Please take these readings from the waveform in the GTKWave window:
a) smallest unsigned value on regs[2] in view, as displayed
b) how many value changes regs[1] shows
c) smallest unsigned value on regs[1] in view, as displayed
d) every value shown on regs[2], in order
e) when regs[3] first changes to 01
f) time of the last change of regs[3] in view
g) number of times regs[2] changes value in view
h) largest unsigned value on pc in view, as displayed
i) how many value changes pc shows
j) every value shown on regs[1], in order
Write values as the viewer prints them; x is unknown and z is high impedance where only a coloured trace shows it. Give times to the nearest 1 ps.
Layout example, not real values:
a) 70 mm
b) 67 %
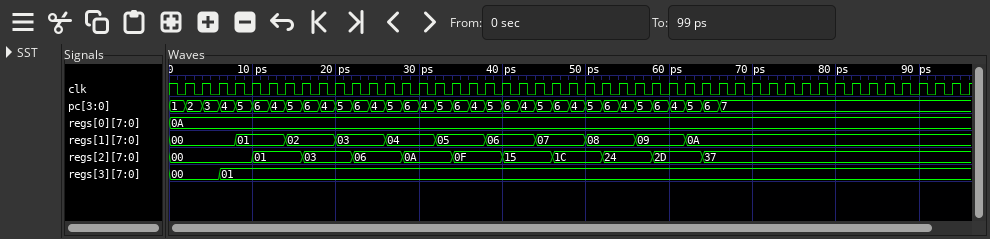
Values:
a) 00
b) 10
c) 00
d) 00, 01, 03, 06, 0A, 0F, 15, 1C, 24, 2D, 37
e) 6 ps
f) 6 ps
g) 10
h) 7
i) 33
j) 00, 01, 02, 03, 04, 05, 06, 07, 08, 09, 0A
